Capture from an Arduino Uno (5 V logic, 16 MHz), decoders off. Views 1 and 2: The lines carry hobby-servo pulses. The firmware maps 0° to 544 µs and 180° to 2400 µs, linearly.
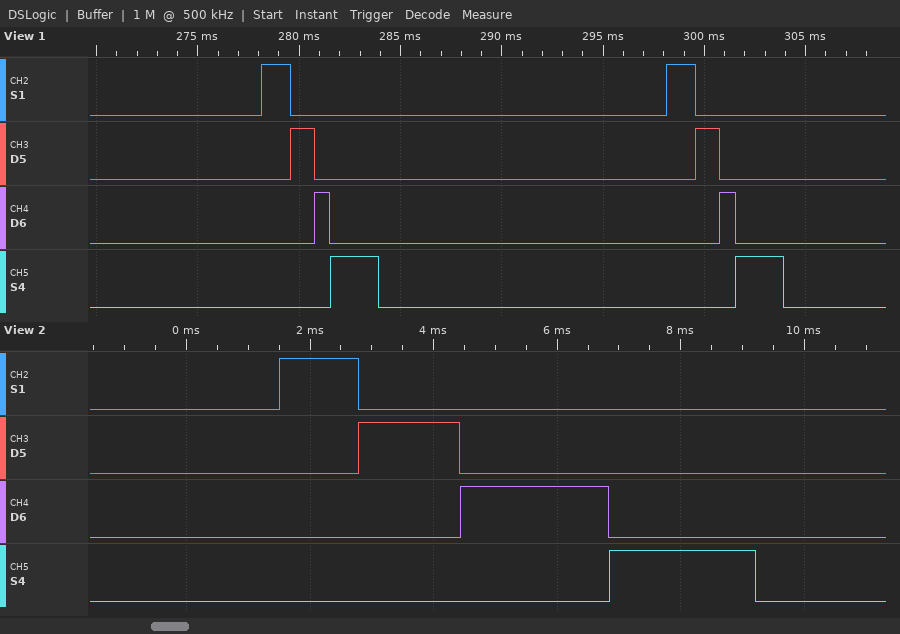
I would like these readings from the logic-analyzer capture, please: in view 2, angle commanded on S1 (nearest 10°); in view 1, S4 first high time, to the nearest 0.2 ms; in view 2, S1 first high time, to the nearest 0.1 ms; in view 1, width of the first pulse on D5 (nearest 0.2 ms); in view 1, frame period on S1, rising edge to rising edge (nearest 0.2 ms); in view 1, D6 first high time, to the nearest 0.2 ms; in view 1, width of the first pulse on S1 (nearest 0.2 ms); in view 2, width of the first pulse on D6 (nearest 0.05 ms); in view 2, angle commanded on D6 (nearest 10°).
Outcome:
70°
2.4 ms
1.3 ms
1.2 ms
20.0 ms
0.8 ms
1.4 ms
2.40 ms
180°
